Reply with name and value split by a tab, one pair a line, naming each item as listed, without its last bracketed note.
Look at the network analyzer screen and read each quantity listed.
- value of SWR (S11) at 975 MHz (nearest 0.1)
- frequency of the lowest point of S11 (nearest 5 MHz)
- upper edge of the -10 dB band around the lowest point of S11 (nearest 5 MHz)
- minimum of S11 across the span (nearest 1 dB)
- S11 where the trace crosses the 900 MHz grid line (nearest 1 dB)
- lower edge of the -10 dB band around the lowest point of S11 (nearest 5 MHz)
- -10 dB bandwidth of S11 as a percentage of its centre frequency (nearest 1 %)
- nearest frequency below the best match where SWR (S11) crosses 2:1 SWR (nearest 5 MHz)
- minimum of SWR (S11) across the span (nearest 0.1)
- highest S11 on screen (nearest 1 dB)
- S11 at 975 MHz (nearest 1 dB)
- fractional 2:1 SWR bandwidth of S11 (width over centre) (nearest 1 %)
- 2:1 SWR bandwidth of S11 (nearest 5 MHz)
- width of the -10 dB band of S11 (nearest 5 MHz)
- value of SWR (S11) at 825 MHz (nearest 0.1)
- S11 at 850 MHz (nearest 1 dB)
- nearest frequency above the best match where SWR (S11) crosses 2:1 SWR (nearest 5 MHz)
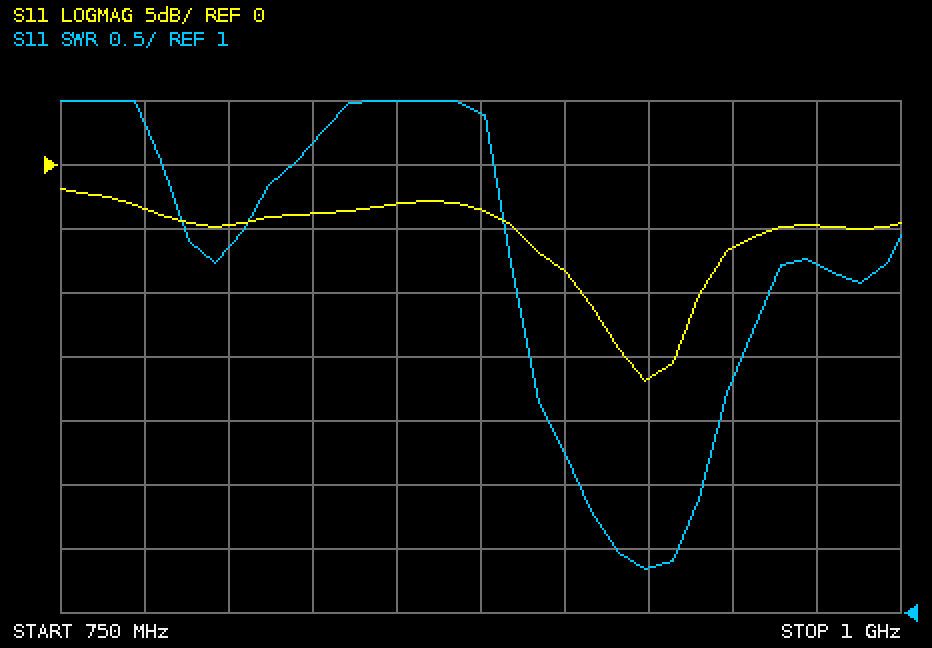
value of SWR (S11) at 975 MHz	3.7
frequency of the lowest point of S11	925 MHz
upper edge of the -10 dB band around the lowest point of S11	940 MHz
minimum of S11 across the span	-17 dB
S11 where the trace crosses the 900 MHz grid line	-8 dB
lower edge of the -10 dB band around the lowest point of S11	905 MHz
-10 dB bandwidth of S11 as a percentage of its centre frequency	4 %
nearest frequency below the best match where SWR (S11) crosses 2:1 SWR	905 MHz
minimum of SWR (S11) across the span	1.3
highest S11 on screen	-2 dB
S11 at 975 MHz	-5 dB
fractional 2:1 SWR bandwidth of S11 (width over centre)	4 %
2:1 SWR bandwidth of S11	35 MHz
width of the -10 dB band of S11	35 MHz
value of SWR (S11) at 825 MHz	4.7
S11 at 850 MHz	-3 dB
nearest frequency above the best match where SWR (S11) crosses 2:1 SWR	940 MHz
